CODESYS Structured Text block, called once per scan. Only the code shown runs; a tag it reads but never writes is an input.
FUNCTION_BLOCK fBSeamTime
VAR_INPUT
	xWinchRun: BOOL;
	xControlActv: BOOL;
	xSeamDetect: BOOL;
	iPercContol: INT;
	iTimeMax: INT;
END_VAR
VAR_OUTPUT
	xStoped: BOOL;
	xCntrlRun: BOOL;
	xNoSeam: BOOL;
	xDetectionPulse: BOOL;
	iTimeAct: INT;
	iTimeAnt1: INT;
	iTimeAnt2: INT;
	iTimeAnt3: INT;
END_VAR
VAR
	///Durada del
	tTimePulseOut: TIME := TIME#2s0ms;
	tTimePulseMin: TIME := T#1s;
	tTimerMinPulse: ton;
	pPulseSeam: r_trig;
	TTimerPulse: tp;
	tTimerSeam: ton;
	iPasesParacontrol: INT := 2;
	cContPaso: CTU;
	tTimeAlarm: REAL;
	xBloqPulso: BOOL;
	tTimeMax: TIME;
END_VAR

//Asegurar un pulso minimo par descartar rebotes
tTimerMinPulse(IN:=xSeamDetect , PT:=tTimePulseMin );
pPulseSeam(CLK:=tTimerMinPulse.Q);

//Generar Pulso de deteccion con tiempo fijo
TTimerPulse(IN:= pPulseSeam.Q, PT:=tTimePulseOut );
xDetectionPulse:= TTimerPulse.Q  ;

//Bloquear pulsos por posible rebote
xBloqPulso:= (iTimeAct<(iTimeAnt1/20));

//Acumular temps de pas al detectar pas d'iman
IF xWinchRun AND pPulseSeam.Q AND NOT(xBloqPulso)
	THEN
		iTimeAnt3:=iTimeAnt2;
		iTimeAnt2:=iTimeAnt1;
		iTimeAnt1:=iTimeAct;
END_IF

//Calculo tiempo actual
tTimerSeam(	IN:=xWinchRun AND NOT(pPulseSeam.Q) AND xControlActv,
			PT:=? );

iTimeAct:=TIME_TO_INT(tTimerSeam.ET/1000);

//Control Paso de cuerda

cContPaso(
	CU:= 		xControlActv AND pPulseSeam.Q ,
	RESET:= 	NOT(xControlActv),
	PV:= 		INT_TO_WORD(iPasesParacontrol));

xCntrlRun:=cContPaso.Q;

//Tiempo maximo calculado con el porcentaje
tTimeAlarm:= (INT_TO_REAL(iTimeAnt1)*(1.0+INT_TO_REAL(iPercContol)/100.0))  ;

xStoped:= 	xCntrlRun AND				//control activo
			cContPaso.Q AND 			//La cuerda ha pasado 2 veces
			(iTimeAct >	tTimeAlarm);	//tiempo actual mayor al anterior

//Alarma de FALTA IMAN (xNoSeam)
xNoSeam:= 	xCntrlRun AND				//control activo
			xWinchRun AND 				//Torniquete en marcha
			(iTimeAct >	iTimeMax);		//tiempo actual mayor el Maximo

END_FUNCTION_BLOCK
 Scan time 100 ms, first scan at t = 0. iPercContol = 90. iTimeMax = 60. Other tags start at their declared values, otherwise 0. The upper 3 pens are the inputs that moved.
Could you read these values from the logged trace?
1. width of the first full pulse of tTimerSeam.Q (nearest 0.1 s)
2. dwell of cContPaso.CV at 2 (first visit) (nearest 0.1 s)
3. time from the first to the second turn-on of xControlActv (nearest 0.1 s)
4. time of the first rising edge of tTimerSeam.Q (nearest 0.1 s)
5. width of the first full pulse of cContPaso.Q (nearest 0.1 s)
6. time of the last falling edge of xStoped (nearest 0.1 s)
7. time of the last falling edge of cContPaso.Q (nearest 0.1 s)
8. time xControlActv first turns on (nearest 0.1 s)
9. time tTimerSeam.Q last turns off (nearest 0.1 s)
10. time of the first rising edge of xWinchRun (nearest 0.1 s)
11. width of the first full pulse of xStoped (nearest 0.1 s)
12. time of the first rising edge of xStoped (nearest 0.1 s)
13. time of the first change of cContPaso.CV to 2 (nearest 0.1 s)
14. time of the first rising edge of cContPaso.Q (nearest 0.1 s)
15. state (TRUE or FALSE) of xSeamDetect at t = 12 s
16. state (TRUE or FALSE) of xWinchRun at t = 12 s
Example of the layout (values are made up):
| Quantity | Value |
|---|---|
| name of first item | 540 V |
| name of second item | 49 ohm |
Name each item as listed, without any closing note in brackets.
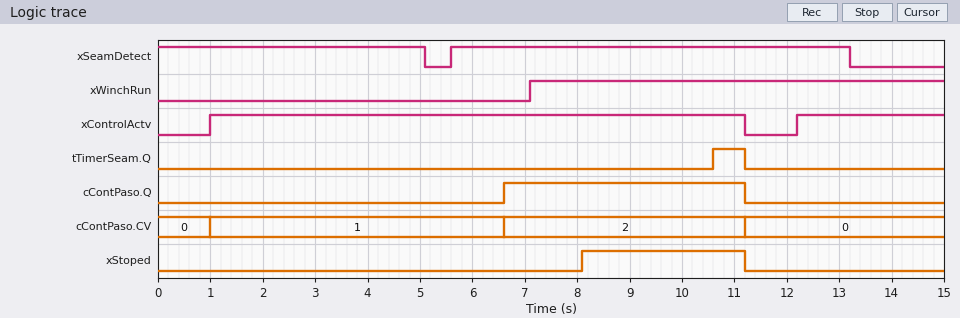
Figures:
| Quantity | Value |
|---|---|
| width of the first full pulse of tTimerSeam.Q | 0.6 s |
| dwell of cContPaso.CV at 2 (first visit) | 4.6 s |
| time from the first to the second turn-on of xControlActv | 11.2 s |
| time of the first rising edge of tTimerSeam.Q | 10.6 s |
| width of the first full pulse of cContPaso.Q | 4.6 s |
| time of the last falling edge of xStoped | 11.2 s |
| time of the last falling edge of cContPaso.Q | 11.2 s |
| time xControlActv first turns on | 1.0 s |
| time tTimerSeam.Q last turns off | 11.2 s |
| time of the first rising edge of xWinchRun | 7.1 s |
| width of the first full pulse of xStoped | 3.1 s |
| time of the first rising edge of xStoped | 8.1 s |
| time of the first change of cContPaso.CV to 2 | 6.6 s |
| time of the first rising edge of cContPaso.Q | 6.6 s |
| state (TRUE or FALSE) of xSeamDetect at t = 12 s | TRUE |
| state (TRUE or FALSE) of xWinchRun at t = 12 s | TRUE |
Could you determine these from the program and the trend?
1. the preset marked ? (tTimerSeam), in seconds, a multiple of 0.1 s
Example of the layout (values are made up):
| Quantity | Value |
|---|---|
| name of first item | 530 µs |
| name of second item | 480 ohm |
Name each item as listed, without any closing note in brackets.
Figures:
| Quantity | Value |
|---|---|
| the preset marked ? (tTimerSeam), in seconds, a multiple of 0.1 s | 3.5 s |
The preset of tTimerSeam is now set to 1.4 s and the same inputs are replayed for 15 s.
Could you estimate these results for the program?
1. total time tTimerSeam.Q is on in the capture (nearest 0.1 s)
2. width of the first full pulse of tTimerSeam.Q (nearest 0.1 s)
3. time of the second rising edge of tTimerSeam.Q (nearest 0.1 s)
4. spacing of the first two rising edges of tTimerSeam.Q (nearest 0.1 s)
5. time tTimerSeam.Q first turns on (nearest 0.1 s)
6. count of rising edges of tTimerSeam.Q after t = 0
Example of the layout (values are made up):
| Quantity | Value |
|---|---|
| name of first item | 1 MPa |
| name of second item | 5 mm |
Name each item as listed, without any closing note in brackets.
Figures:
| Quantity | Value |
|---|---|
| total time tTimerSeam.Q is on in the capture | 4.1 s |
| width of the first full pulse of tTimerSeam.Q | 2.7 s |
| time of the second rising edge of tTimerSeam.Q | 13.6 s |
| spacing of the first two rising edges of tTimerSeam.Q | 5.1 s |
| time tTimerSeam.Q first turns on | 8.5 s |
| count of rising edges of tTimerSeam.Q after t = 0 | 2 |
